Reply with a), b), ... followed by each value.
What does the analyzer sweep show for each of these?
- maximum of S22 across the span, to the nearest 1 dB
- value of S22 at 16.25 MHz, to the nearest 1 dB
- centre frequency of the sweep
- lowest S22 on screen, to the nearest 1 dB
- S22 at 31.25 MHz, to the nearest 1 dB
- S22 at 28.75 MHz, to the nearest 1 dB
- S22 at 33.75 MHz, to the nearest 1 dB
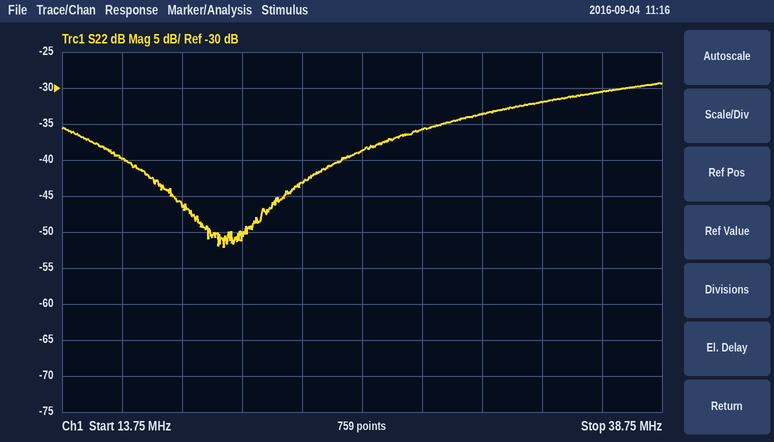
a) -29 dB
b) -40 dB
c) 26.25 MHz
d) -52 dB
e) -34 dB
f) -36 dB
g) -32 dB
